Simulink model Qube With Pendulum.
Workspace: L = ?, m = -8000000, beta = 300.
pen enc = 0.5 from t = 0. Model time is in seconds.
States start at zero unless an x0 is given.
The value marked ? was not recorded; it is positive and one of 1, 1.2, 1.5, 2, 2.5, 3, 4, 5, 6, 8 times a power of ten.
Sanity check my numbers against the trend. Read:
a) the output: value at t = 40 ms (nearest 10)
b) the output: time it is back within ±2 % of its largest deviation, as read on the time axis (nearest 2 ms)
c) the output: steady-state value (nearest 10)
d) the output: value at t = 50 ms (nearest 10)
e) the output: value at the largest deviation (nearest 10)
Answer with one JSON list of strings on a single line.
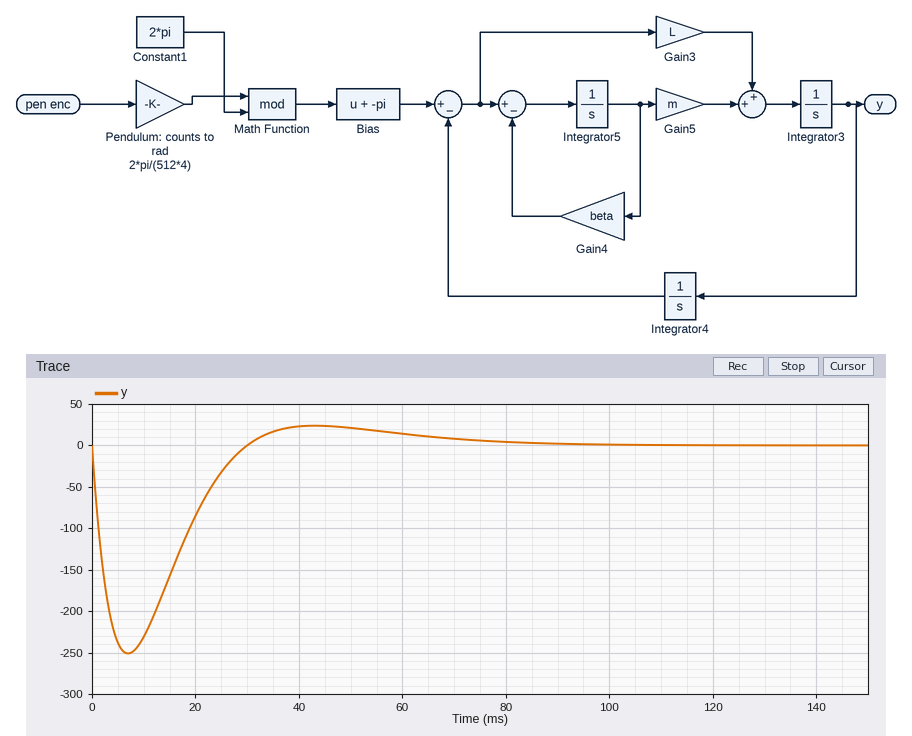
["20", "78 ms", "0", "20", "-250"]
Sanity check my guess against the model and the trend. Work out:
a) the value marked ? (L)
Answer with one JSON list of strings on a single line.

["30000"]
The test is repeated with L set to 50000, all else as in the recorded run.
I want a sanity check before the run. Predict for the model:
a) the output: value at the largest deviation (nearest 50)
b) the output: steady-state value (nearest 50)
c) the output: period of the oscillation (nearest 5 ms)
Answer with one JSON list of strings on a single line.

["-500", "0", "35 ms"]
